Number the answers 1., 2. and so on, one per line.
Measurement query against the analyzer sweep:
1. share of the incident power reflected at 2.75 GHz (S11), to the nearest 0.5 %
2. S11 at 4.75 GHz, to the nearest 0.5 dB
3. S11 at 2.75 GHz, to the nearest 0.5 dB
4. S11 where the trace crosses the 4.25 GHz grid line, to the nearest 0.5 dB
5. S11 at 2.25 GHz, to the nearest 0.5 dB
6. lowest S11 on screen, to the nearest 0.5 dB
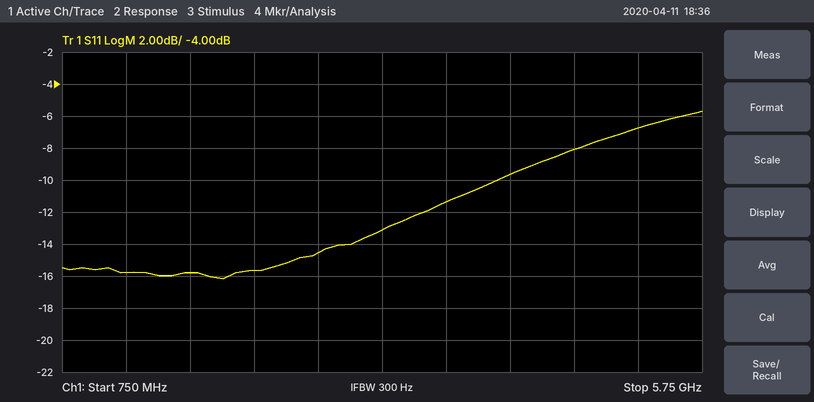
1. 3.5 %
2. -8.0 dB
3. -14.5 dB
4. -9.5 dB
5. -15.5 dB
6. -16.0 dB
